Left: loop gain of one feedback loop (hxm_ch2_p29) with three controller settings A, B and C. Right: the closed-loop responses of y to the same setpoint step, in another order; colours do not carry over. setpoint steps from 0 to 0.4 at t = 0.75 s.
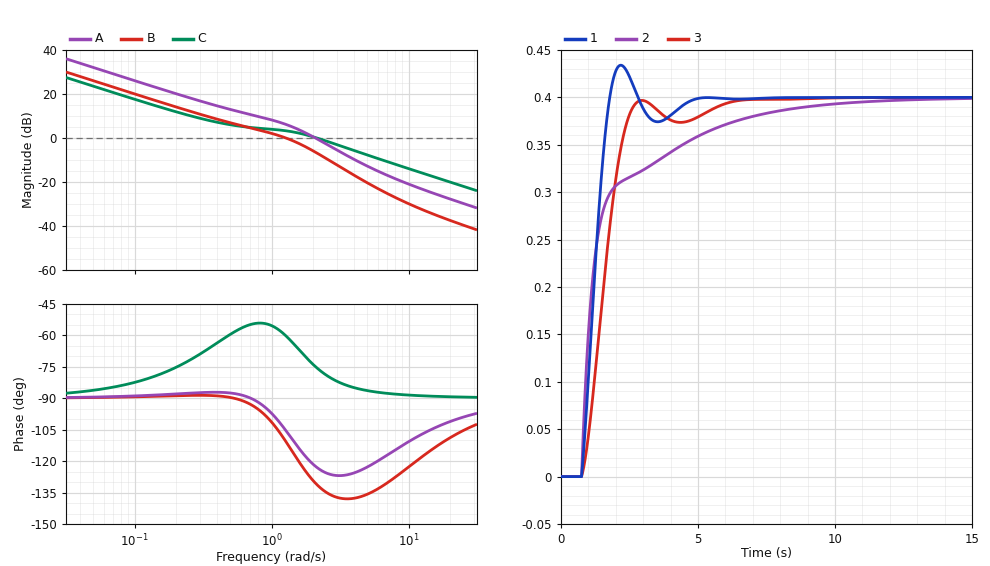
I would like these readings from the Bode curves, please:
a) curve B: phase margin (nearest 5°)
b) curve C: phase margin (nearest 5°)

70°
105°
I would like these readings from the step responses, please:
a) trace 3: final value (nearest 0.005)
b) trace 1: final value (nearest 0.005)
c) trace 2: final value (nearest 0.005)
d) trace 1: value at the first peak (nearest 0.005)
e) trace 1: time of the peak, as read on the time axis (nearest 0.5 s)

0.400
0.400
0.400
0.435
2.0 s
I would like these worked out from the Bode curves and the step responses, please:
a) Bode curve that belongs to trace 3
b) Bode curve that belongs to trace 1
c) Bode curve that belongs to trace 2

B
A
C
